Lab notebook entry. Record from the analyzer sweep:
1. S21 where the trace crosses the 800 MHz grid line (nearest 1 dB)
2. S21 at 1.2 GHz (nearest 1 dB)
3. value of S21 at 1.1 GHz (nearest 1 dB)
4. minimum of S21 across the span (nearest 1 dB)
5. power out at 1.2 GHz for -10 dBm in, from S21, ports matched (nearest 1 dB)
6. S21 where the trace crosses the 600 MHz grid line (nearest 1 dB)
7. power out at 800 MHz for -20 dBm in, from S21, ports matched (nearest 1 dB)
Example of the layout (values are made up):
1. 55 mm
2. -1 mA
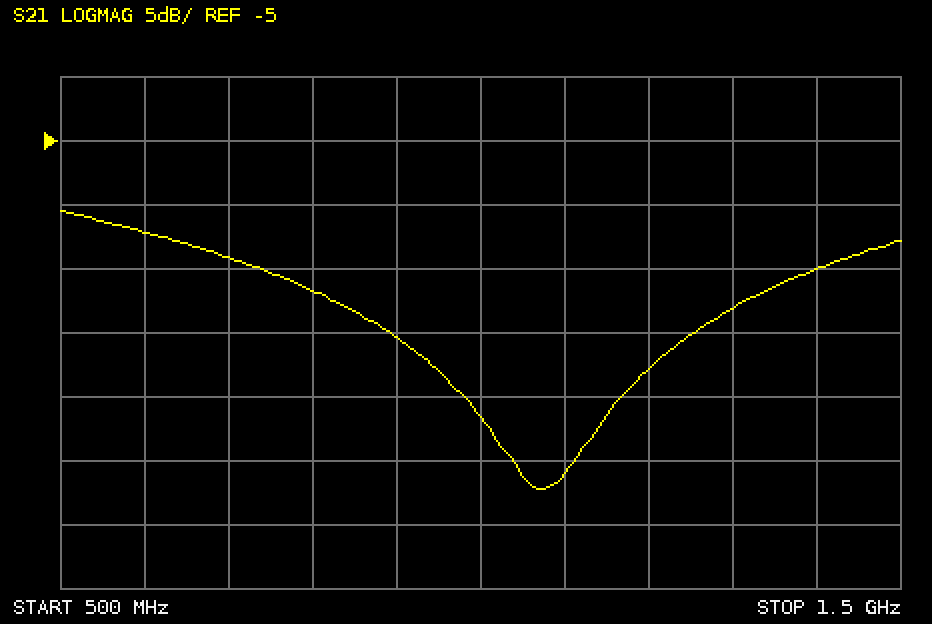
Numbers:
1. -17 dB
2. -23 dB
3. -31 dB
4. -32 dB
5. -33 dBm
6. -12 dB
7. -37 dBm
